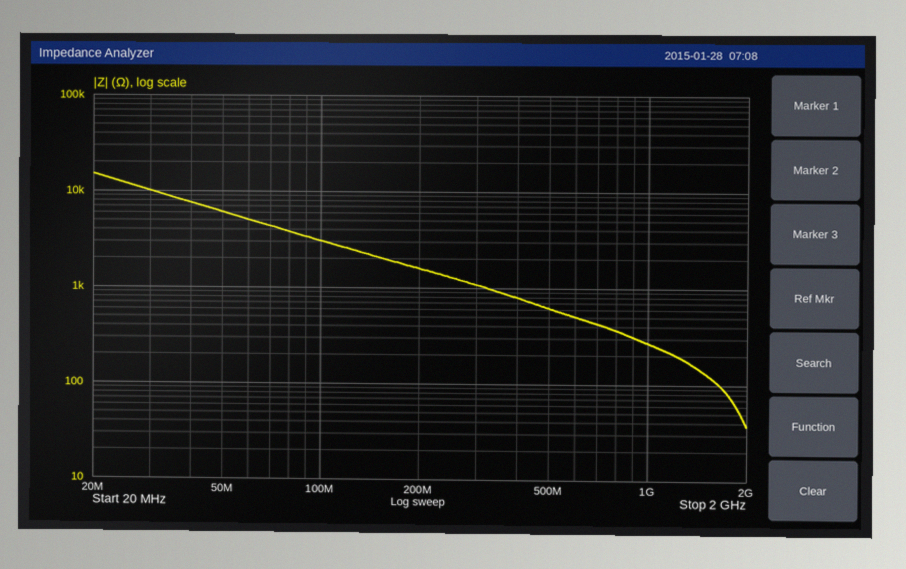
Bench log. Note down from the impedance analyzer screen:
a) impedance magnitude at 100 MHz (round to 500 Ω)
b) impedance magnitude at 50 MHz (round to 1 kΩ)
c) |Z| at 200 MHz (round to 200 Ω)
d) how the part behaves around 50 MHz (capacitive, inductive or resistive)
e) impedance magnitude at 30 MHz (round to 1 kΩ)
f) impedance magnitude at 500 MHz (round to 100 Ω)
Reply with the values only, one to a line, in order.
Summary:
3.0 kΩ
6 kΩ
1.6 kΩ
capacitive
10 kΩ
600 Ω
